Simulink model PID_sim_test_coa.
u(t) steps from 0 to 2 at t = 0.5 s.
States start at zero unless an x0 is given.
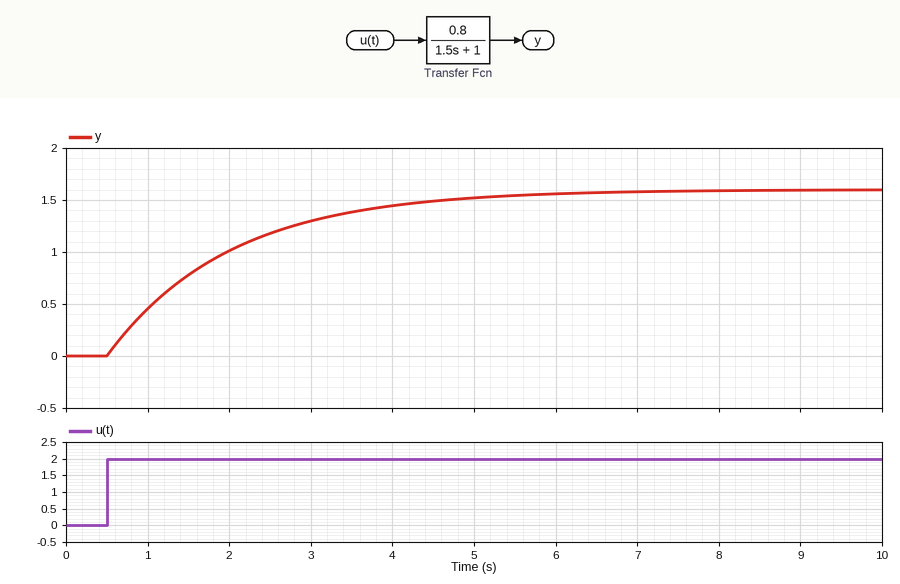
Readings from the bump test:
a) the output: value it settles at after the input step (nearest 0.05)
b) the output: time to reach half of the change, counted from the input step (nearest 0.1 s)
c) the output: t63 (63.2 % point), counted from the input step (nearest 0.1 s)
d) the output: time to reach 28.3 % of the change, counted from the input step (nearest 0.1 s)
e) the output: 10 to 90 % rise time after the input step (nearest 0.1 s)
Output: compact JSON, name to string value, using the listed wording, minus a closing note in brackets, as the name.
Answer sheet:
{"the output: value it settles at after the input step": "1.60", "the output: time to reach half of the change, counted from the input step": "1.0 s", "the output: t63 (63.2 % point), counted from the input step": "1.5 s", "the output: time to reach 28.3 % of the change, counted from the input step": "0.5 s", "the output: 10 to 90 % rise time after the input step": "3.3 s"}
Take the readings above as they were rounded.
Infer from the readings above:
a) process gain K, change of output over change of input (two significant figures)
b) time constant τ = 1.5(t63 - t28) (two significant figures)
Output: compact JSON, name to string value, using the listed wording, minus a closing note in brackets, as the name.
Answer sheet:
{"process gain K, change of output over change of input": "0.80", "time constant τ = 1.5(t63 - t28)": "1.5 s"}
